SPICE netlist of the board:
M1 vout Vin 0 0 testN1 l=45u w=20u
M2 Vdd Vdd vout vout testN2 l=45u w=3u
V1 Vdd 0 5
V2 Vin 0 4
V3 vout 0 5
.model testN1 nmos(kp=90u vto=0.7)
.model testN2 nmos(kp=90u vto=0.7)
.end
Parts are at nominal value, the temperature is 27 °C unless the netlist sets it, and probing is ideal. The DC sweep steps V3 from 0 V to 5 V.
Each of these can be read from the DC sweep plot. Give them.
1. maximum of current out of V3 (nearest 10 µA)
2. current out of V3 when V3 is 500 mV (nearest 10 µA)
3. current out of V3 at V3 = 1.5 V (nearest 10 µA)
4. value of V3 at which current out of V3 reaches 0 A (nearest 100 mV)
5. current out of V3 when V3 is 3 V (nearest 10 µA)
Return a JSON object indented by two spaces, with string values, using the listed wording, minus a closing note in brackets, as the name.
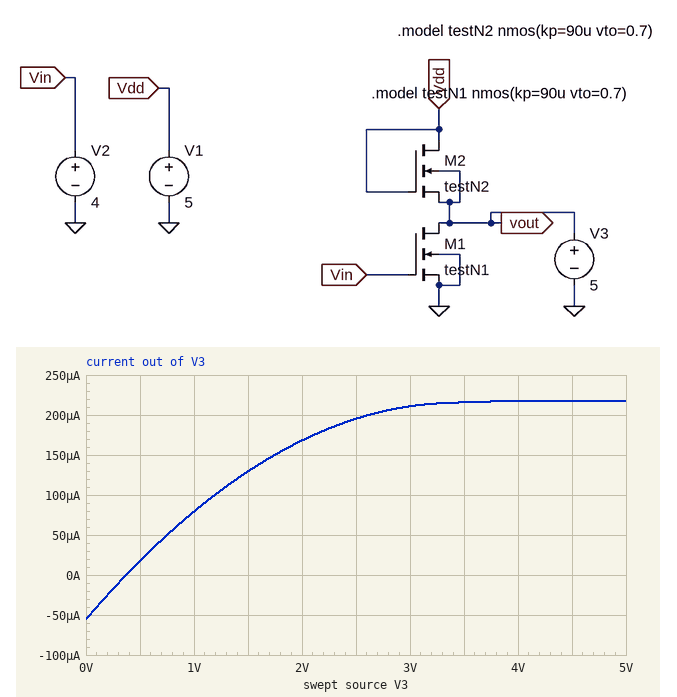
{
  "maximum of current out of V3": "220 µA",
  "current out of V3 when V3 is 500 mV": "20 µA",
  "current out of V3 at V3 = 1.5 V": "130 µA",
  "value of V3 at which current out of V3 reaches 0 A": "400 mV",
  "current out of V3 when V3 is 3 V": "210 µA"
}
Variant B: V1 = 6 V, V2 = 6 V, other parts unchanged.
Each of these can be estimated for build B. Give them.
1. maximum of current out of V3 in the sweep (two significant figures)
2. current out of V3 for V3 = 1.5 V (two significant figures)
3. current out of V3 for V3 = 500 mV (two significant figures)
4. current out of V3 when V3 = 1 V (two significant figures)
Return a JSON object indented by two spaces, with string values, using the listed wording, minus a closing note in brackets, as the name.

{
  "maximum of current out of V3 in the sweep": "560 µA",
  "current out of V3 for V3 = 1.5 V": "230 µA",
  "current out of V3 for V3 = 500 mV": "32 µA",
  "current out of V3 when V3 = 1 V": "140 µA"
}
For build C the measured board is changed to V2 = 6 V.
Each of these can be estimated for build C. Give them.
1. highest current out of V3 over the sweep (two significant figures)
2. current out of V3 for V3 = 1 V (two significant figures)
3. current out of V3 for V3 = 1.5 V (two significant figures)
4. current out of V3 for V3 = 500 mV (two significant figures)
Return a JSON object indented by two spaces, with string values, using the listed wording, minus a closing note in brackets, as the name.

{
  "highest current out of V3 over the sweep": "560 µA",
  "current out of V3 for V3 = 1 V": "160 µA",
  "current out of V3 for V3 = 1.5 V": "250 µA",
  "current out of V3 for V3 = 500 mV": "58 µA"
}
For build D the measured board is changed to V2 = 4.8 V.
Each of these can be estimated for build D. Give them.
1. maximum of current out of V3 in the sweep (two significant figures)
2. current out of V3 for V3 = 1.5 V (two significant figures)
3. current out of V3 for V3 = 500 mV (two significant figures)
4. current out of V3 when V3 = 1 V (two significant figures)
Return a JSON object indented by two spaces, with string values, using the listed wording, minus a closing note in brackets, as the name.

{
  "maximum of current out of V3 in the sweep": "340 µA",
  "current out of V3 for V3 = 1.5 V": "180 µA",
  "current out of V3 for V3 = 500 mV": "34 µA",
  "current out of V3 when V3 = 1 V": "110 µA"
}
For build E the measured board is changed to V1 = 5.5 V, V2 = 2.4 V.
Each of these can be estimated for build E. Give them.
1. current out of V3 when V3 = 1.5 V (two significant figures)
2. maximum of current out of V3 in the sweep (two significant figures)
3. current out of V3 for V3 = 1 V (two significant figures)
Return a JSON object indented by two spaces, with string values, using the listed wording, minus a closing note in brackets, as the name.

{
  "current out of V3 when V3 = 1.5 V": "24 µA",
  "maximum of current out of V3 in the sweep": "58 µA",
  "current out of V3 for V3 = 1 V": "4.7 µA"
}
